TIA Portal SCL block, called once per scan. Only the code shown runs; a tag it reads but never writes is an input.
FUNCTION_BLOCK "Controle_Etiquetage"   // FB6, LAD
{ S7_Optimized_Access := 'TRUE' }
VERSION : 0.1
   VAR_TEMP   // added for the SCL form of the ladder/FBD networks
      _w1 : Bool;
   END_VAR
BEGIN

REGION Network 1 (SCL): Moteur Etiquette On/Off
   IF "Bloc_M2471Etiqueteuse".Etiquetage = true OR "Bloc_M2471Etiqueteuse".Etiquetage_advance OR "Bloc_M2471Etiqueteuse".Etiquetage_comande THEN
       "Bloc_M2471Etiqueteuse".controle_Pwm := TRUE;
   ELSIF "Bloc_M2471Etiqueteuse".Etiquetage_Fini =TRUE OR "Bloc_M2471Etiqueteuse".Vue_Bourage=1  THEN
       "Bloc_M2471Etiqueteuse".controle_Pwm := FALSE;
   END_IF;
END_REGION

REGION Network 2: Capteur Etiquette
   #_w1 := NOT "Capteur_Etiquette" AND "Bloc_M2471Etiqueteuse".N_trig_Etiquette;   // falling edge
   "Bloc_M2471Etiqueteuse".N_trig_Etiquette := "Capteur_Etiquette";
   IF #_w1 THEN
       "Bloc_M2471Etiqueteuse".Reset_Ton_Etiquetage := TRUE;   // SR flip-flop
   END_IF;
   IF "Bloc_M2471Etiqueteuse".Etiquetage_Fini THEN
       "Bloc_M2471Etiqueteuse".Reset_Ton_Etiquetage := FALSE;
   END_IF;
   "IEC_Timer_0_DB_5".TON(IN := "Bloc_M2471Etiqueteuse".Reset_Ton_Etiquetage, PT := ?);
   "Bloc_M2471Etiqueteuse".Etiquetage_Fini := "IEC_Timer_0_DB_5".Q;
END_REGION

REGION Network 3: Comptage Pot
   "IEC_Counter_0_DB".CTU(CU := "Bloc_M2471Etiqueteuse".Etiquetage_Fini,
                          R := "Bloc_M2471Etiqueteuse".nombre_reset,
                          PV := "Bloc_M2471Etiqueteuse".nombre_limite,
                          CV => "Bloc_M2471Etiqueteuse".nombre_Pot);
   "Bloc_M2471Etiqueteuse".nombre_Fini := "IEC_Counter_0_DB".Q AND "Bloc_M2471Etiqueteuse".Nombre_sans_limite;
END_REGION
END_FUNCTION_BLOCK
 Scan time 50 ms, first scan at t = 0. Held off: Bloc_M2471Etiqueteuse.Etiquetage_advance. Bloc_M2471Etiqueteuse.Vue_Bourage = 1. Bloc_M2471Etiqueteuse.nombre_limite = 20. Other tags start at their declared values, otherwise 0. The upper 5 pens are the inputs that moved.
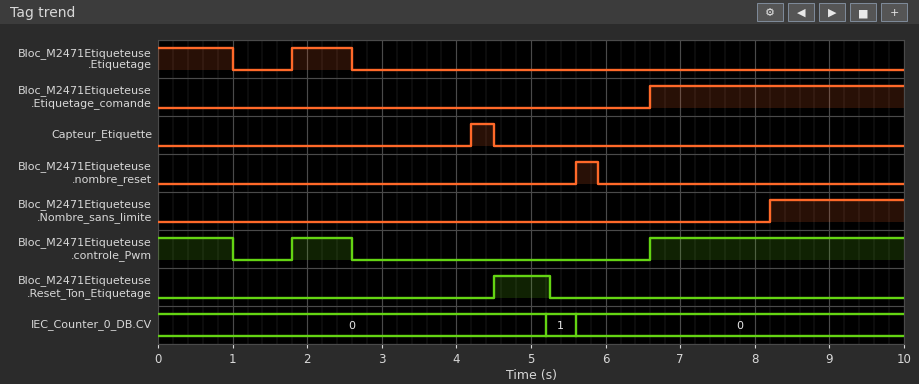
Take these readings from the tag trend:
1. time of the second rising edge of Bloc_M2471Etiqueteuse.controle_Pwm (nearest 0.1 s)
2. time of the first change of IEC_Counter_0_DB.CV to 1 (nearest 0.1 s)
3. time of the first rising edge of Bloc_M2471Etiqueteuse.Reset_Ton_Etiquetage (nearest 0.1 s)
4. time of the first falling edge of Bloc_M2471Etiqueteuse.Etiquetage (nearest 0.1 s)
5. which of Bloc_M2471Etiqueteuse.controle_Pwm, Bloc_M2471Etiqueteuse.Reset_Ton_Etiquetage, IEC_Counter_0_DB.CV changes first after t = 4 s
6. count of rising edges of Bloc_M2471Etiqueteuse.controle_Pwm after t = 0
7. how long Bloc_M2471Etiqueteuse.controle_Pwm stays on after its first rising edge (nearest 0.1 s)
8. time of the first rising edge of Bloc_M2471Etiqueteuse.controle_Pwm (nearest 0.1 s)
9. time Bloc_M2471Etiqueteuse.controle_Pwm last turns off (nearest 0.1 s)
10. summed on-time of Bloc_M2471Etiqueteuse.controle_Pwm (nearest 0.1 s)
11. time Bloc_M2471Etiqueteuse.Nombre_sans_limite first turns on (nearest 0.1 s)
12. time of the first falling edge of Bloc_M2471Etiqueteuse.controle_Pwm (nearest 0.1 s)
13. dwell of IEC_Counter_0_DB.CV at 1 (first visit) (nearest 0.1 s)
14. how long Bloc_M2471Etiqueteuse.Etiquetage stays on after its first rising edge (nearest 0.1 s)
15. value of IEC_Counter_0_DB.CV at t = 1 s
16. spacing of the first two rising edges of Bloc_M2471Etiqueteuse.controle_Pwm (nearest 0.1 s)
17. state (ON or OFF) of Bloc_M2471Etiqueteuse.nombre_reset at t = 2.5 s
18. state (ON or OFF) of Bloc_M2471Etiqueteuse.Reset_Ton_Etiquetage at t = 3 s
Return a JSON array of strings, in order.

["6.6 s", "5.2 s", "4.5 s", "1.0 s", "Bloc_M2471Etiqueteuse.Reset_Ton_Etiquetage", "2", "0.8 s", "1.8 s", "2.6 s", "5.2 s", "8.2 s", "1.0 s", "0.4 s", "0.8 s", "0", "4.8 s", "OFF", "OFF"]
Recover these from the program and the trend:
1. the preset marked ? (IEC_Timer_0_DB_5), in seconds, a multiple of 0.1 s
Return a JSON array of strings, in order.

["0.7 s"]
